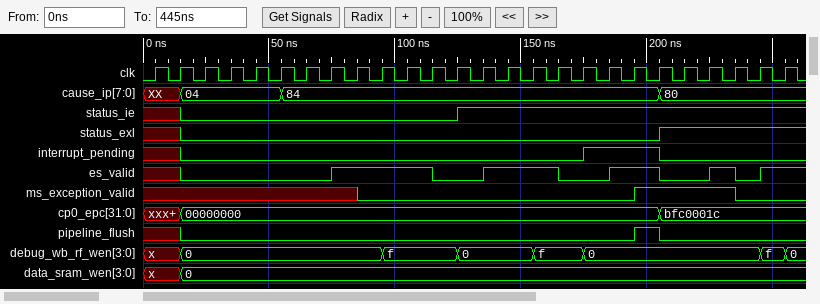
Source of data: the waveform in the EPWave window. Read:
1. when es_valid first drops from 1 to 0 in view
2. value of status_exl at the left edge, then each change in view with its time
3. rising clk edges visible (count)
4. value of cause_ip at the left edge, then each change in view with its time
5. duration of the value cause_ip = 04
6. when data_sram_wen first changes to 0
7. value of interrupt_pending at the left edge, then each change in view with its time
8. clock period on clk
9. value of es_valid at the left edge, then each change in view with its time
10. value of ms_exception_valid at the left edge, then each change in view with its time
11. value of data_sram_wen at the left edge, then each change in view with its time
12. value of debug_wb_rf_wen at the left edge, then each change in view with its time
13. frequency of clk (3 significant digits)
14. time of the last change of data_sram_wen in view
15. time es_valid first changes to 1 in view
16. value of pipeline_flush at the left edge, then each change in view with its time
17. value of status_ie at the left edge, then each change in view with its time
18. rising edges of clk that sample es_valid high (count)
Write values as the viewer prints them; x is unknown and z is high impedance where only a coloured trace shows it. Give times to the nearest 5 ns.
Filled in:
115 ns
x, 0 at 15 ns, 1 at 205 ns
26
XX, 04 at 15 ns, 84 at 55 ns, 80 at 205 ns
40 ns
15 ns
x, 0 at 15 ns, 1 at 175 ns, 0 at 205 ns
10 ns
x, 0 at 15 ns, 1 at 75 ns, 0 at 115 ns, 1 at 135 ns, 0 at 165 ns, 1 at 185 ns, 0 at 205 ns, 1 at 225 ns, 0 at 235 ns, 1 at 245 ns
x, 0 at 85 ns, 1 at 195 ns, 0 at 235 ns
x, 0 at 15 ns
x, 0 at 15 ns, f at 95 ns, 0 at 125 ns, f at 155 ns, 0 at 175 ns, f at 245 ns, 0 at 255 ns
100 MHz
15 ns
75 ns
x, 0 at 15 ns, 1 at 195 ns, 0 at 205 ns
x, 0 at 15 ns, 1 at 125 ns
11
